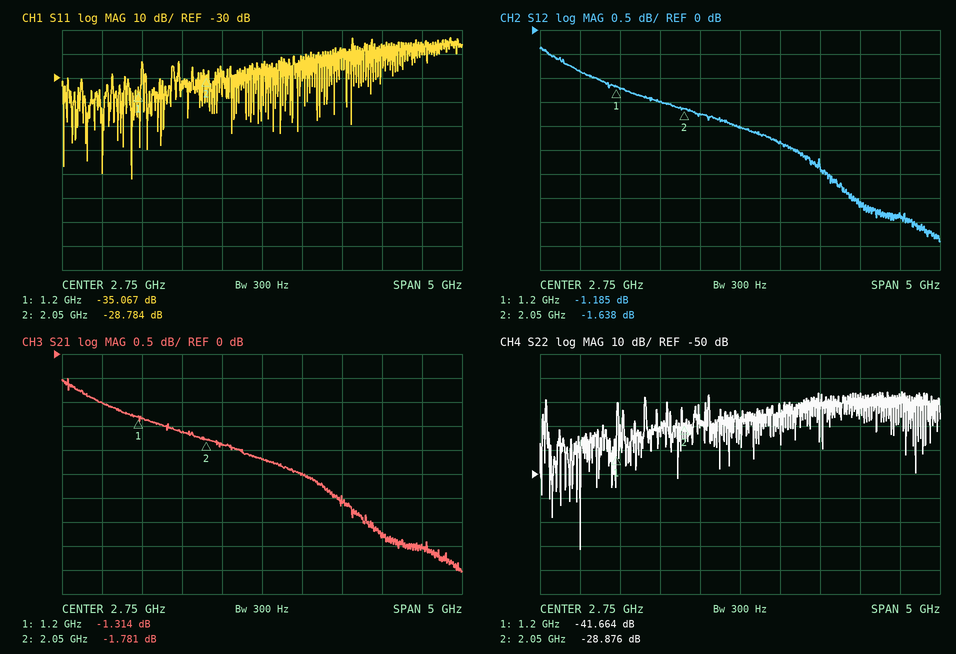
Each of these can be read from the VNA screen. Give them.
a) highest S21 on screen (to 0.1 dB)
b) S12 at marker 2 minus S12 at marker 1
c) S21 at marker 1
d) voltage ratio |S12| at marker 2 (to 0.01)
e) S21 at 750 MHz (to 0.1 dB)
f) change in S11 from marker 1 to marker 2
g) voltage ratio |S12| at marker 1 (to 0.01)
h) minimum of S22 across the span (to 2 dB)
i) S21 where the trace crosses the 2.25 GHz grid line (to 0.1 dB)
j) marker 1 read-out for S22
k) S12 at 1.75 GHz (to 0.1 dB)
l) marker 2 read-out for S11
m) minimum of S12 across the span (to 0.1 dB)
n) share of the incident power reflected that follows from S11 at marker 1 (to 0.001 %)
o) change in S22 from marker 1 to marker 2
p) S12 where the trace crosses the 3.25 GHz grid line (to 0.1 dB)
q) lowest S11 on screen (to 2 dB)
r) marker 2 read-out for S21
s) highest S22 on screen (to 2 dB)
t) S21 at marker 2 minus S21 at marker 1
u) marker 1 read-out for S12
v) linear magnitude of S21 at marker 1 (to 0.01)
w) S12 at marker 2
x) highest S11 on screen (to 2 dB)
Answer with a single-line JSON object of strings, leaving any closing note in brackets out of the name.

{"highest S21 on screen": "-0.5 dB", "S12 at marker 2 minus S12 at marker 1": "-0.453 dB", "S21 at marker 1": "-1.314 dB", "voltage ratio |S12| at marker 2": "0.83", "S21 at 750 MHz": "-1.0 dB", "change in S11 from marker 1 to marker 2": "6.283 dB", "voltage ratio |S12| at marker 1": "0.87", "minimum of S22 across the span": "-82 dB", "S21 where the trace crosses the 2.25 GHz grid line": "-1.9 dB", "marker 1 read-out for S22": "-41.664 dB", "S12 at 1.75 GHz": "-1.5 dB", "marker 2 read-out for S11": "-28.784 dB", "minimum of S12 across the span": "-4.4 dB", "share of the incident power reflected that follows from S11 at marker 1": "0.031 %", "change in S22 from marker 1 to marker 2": "12.788 dB", "S12 where the trace crosses the 3.25 GHz grid line": "-2.3 dB", "lowest S11 on screen": "-72 dB", "marker 2 read-out for S21": "-1.781 dB", "highest S22 on screen": "-16 dB", "S21 at marker 2 minus S21 at marker 1": "-0.467 dB", "marker 1 read-out for S12": "-1.185 dB", "linear magnitude of S21 at marker 1": "0.86", "S12 at marker 2": "-1.638 dB", "highest S11 on screen": "-14 dB"}
